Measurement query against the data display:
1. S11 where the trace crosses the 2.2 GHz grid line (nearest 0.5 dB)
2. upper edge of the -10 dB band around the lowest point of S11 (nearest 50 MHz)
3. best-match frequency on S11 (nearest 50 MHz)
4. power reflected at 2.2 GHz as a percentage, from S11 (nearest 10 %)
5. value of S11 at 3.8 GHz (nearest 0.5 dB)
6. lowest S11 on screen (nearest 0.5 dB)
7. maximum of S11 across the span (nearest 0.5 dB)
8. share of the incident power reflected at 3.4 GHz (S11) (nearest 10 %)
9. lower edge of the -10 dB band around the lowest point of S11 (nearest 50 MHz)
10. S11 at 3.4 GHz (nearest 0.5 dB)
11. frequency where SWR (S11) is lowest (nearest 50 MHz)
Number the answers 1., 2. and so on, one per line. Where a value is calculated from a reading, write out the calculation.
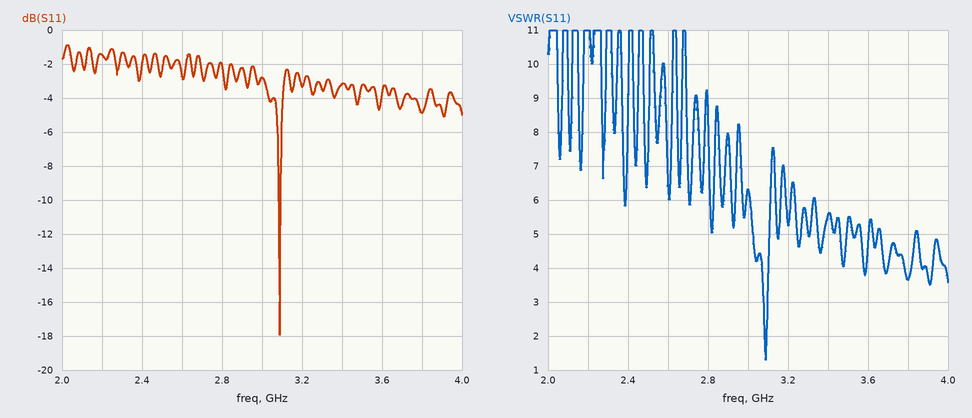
1. -1.5 dB
2. 3.10 GHz
3. 3.10 GHz
4. 10^(-1.5/10) ≈ 70.8 %, so 70 % to the nearest 10 %
5. -5.0 dB
6. -18.0 dB
7. -1.0 dB
8. 10^(-3/10) ≈ 50 %
9. 3.10 GHz
10. -3.0 dB
11. 3.10 GHz
